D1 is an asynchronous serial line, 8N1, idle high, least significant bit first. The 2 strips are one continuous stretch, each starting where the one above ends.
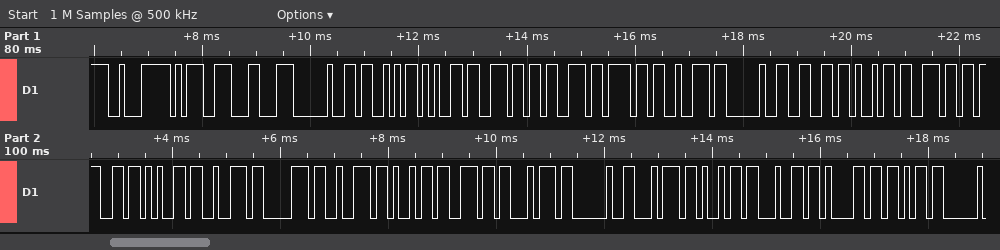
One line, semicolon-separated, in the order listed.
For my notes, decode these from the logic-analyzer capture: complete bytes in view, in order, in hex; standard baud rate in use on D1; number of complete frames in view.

E2 9D 8C 20 53 65 6E 73 6F 72 20 66 69 6E 67 65 72 70 72 69 6E 74 20 74 69 64 61 6B; 9600 baud; 28
